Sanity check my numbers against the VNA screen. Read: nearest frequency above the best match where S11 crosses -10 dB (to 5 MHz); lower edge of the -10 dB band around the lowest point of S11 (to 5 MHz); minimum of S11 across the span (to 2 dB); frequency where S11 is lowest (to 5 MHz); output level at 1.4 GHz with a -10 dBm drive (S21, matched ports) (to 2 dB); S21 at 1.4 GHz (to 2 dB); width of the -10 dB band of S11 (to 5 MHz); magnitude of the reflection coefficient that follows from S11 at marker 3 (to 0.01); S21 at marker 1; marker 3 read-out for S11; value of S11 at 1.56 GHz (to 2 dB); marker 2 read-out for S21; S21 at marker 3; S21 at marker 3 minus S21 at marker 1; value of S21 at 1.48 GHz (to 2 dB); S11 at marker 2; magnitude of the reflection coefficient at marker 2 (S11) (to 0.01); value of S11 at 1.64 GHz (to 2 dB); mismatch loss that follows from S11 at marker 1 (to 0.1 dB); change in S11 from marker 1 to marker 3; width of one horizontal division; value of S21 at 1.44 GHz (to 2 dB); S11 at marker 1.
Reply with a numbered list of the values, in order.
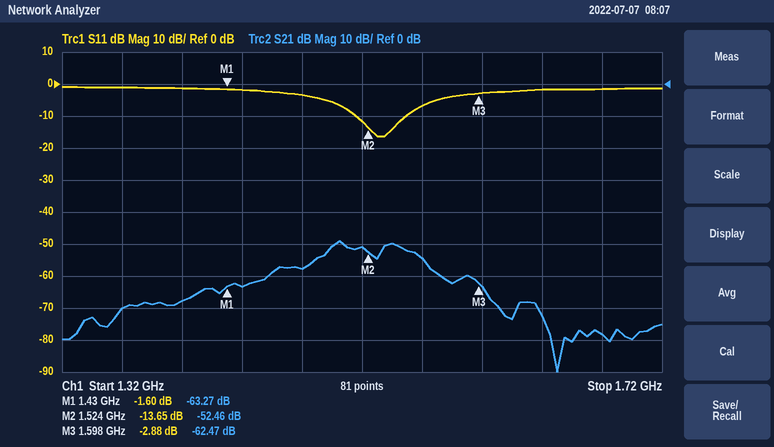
1. 1.550 GHz
2. 1.515 GHz
3. -16 dB
4. 1.530 GHz
5. -78 dBm
6. -68 dB
7. 35 MHz
8. 0.72
9. -63.27 dB
10. -2.88 dB
11. -6 dB
12. -52.46 dB
13. -62.47 dB
14. 0.80 dB
15. -58 dB
16. -13.65 dB
17. 0.21
18. -2 dB
19. 5.1 dB
20. -1.28 dB
21. 40 MHz
22. -64 dB
23. -1.60 dB
